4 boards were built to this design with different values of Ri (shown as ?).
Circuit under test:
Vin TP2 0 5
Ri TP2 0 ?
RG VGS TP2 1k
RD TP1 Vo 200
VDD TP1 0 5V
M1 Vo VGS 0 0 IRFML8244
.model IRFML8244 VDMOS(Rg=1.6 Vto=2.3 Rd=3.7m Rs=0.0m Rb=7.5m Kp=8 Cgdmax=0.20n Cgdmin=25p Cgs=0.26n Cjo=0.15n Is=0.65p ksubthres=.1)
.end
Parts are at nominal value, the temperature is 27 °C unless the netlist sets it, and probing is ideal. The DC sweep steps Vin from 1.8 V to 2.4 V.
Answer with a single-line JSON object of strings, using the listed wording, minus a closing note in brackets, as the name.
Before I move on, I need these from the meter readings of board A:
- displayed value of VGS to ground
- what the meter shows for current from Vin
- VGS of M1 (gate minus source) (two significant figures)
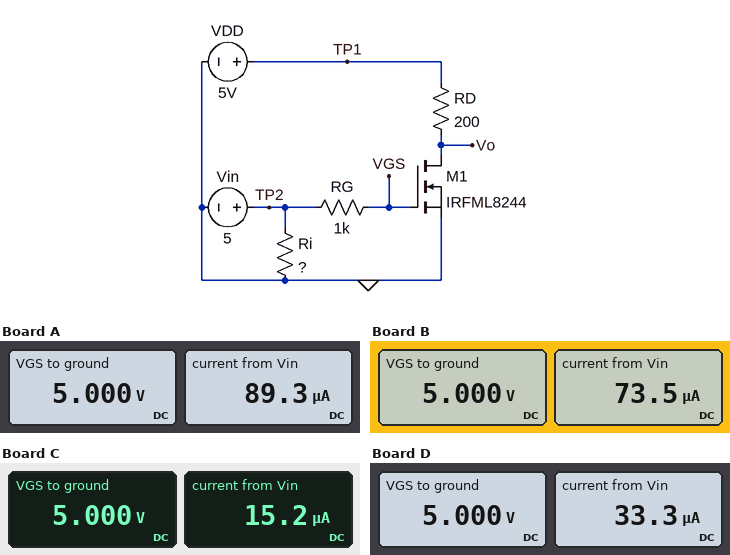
{"displayed value of VGS to ground": "5.000 V", "what the meter shows for current from Vin": "89.3 µA", "VGS of M1 (gate minus source)": "5.0 V"}
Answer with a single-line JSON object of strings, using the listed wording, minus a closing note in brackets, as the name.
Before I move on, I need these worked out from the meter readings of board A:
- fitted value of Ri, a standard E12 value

{"fitted value of Ri, a standard E12 value": "56 kΩ"}
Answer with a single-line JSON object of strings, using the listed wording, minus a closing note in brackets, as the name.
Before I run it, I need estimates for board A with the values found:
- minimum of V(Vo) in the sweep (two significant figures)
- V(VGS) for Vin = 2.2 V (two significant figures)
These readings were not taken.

{"minimum of V(Vo) in the sweep": "26 mV", "V(VGS) for Vin = 2.2 V": "2.2 V"}
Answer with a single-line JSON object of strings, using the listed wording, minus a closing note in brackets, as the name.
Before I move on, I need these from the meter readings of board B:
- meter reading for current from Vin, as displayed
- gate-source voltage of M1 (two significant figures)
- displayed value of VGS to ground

{"meter reading for current from Vin, as displayed": "73.5 µA", "gate-source voltage of M1": "5.0 V", "displayed value of VGS to ground": "5.000 V"}
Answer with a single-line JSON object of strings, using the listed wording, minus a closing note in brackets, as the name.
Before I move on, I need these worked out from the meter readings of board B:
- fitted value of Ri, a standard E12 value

{"fitted value of Ri, a standard E12 value": "68 kΩ"}
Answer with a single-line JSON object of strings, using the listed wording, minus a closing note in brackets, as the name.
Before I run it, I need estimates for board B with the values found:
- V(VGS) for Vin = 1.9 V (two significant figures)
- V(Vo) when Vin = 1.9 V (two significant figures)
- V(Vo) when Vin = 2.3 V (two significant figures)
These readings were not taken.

{"V(VGS) for Vin = 1.9 V": "1.9 V", "V(Vo) when Vin = 1.9 V": "5.0 V", "V(Vo) when Vin = 2.3 V": "1.2 V"}
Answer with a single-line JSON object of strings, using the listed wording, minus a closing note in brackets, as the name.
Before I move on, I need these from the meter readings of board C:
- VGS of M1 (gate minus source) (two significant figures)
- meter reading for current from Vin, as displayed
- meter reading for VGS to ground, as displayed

{"VGS of M1 (gate minus source)": "5.0 V", "meter reading for current from Vin, as displayed": "15.2 µA", "meter reading for VGS to ground, as displayed": "5.000 V"}
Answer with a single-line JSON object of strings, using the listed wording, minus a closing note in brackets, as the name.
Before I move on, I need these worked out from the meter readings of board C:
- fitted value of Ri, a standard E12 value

{"fitted value of Ri, a standard E12 value": "330 kΩ"}
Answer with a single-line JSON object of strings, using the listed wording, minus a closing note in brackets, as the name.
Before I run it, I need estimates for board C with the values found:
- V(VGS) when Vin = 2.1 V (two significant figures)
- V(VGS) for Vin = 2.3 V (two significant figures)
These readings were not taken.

{"V(VGS) when Vin = 2.1 V": "2.1 V", "V(VGS) for Vin = 2.3 V": "2.3 V"}
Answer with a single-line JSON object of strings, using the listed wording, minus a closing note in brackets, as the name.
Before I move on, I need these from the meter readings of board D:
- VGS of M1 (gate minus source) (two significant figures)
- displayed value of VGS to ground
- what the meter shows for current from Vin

{"VGS of M1 (gate minus source)": "5.0 V", "displayed value of VGS to ground": "5.000 V", "what the meter shows for current from Vin": "33.3 µA"}
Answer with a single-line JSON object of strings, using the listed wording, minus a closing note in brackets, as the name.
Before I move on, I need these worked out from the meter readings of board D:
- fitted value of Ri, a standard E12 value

{"fitted value of Ri, a standard E12 value": "150 kΩ"}
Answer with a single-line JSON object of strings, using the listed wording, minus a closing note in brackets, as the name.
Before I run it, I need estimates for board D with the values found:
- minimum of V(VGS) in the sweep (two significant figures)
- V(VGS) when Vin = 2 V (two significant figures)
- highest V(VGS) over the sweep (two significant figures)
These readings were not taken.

{"minimum of V(VGS) in the sweep": "1.8 V", "V(VGS) when Vin = 2 V": "2.0 V", "highest V(VGS) over the sweep": "2.4 V"}
